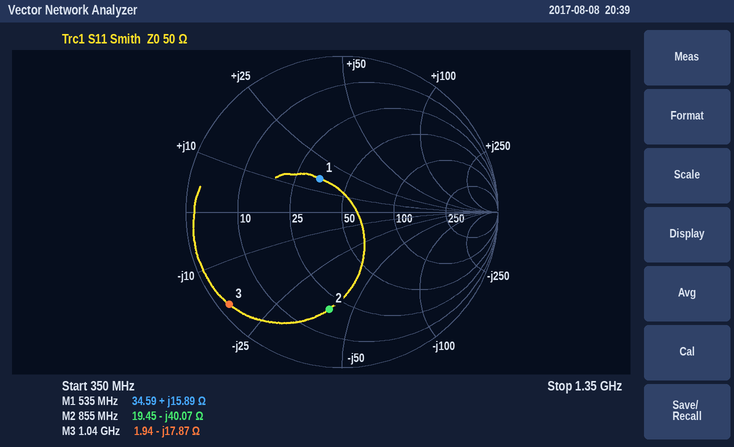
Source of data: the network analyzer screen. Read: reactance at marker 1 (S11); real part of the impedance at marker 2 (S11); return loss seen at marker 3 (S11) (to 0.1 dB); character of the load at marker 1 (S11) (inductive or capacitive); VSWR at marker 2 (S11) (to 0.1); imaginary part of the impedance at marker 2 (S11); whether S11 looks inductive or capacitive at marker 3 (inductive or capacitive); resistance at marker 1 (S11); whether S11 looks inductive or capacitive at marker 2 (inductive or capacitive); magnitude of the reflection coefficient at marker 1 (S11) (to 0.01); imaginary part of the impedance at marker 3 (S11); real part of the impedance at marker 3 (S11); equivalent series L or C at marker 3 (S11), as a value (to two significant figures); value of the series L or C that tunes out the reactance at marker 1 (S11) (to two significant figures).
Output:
+15.89 Ω
19.45 Ω
0.6 dB
inductive
4.4
-40.07 Ω
capacitive
34.59 Ω
capacitive
0.26
-17.87 Ω
1.94 Ω
8.6 pF
19 pF
